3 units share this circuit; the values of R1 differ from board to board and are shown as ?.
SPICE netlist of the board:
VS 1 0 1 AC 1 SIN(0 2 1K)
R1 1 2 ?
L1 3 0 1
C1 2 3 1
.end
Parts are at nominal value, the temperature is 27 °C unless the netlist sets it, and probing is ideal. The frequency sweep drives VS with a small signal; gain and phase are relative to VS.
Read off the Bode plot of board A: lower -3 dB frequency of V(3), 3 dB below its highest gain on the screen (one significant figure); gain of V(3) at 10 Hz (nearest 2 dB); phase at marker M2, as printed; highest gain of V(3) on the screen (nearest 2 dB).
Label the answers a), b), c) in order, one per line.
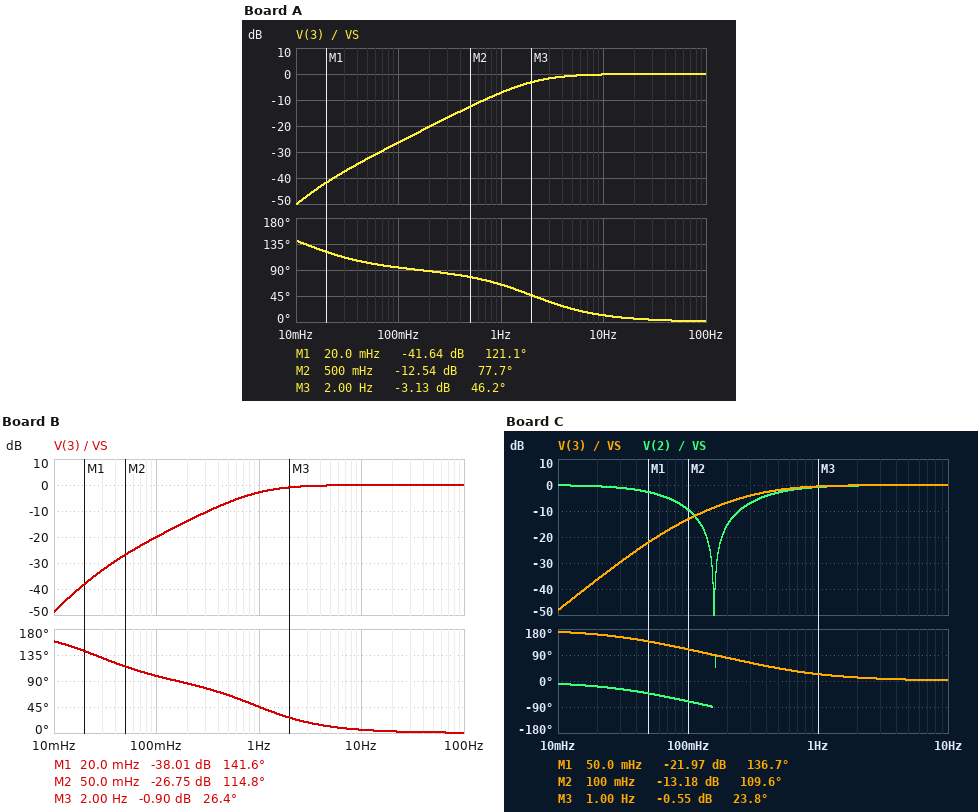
a) 2 Hz
b) 0 dB
c) 77.7 deg
d) 0 dB
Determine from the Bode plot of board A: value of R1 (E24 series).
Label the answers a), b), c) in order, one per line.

a) 13 Ω
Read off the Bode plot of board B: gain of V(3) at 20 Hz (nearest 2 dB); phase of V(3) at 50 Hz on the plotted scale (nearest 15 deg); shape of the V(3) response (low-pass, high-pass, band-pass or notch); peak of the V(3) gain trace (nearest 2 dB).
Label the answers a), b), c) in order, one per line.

a) 0 dB
b) 0 deg
c) high-pass
d) 0 dB
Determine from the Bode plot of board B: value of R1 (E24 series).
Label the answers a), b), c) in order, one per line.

a) 6.2 Ω
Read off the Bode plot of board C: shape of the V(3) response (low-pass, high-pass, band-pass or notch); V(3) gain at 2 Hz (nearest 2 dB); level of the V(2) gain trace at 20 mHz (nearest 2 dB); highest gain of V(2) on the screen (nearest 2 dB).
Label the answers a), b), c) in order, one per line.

a) high-pass
b) 0 dB
c) 0 dB
d) 0 dB
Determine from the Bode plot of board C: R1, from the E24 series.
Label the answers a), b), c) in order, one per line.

a) 2.7 Ω
